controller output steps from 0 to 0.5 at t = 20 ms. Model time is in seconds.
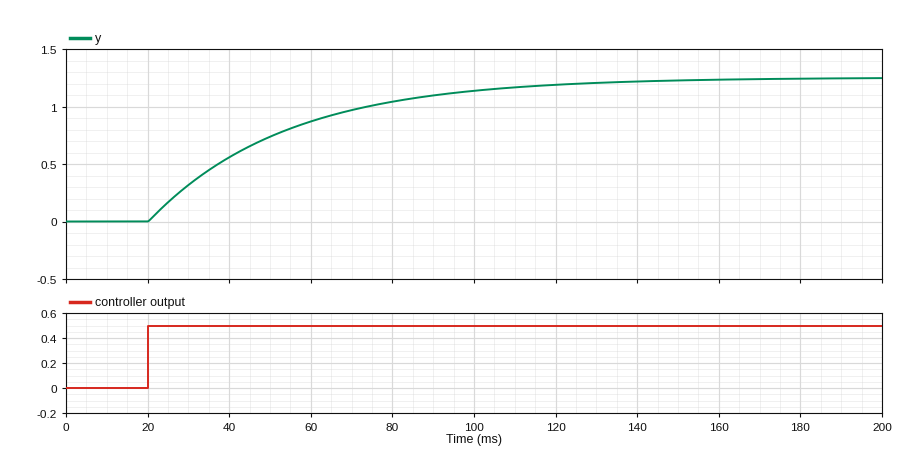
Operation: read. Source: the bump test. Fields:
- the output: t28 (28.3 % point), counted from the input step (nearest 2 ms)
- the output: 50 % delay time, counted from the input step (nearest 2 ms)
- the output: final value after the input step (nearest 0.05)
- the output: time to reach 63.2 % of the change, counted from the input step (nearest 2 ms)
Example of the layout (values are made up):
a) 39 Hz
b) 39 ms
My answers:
a) 12 ms
b) 24 ms
c) 1.25
d) 34 ms
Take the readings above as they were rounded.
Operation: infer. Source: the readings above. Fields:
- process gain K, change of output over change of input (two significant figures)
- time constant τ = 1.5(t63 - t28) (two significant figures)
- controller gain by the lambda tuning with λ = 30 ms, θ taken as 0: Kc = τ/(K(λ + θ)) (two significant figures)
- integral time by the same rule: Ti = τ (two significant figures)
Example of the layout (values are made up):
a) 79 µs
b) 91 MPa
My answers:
a) 2.5
b) 33 ms
c) 0.44
d) 33 ms
